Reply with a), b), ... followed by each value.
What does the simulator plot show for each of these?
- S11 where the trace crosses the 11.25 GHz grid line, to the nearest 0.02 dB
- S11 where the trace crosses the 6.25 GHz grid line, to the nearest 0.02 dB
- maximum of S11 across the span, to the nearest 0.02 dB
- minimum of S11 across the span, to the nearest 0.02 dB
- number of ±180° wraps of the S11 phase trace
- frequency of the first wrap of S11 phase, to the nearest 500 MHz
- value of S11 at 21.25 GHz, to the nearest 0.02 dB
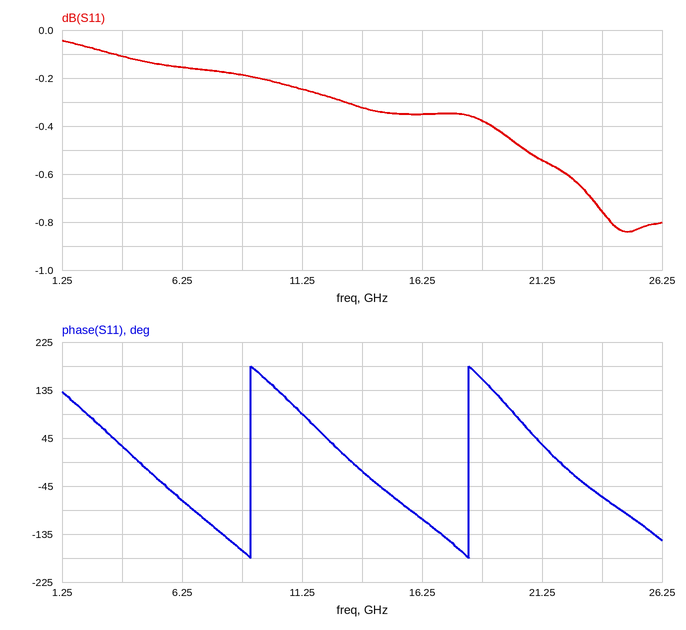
a) -0.24 dB
b) -0.16 dB
c) -0.04 dB
d) -0.84 dB
e) 2
f) 9.0 GHz
g) -0.54 dB
